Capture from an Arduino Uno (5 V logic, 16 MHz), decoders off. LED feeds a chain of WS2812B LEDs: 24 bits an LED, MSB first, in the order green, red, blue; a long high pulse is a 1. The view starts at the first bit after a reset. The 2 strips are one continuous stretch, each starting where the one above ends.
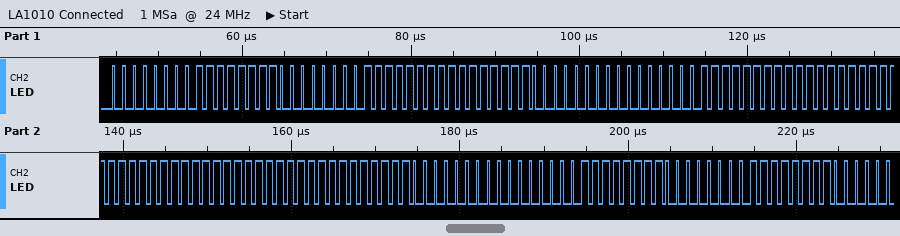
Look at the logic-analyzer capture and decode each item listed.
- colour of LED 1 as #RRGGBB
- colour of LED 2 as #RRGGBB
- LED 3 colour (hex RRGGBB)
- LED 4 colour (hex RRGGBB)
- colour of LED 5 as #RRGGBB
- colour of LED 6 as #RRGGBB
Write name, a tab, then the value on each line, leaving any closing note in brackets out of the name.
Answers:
colour of LED 1 as #RRGGBB	#FF0000
colour of LED 2 as #RRGGBB	#FFFF00
LED 3 colour	#FF00FF
LED 4 colour	#FFFFFF
colour of LED 5 as #RRGGBB	#00FF00
colour of LED 6 as #RRGGBB	#00FFFF
